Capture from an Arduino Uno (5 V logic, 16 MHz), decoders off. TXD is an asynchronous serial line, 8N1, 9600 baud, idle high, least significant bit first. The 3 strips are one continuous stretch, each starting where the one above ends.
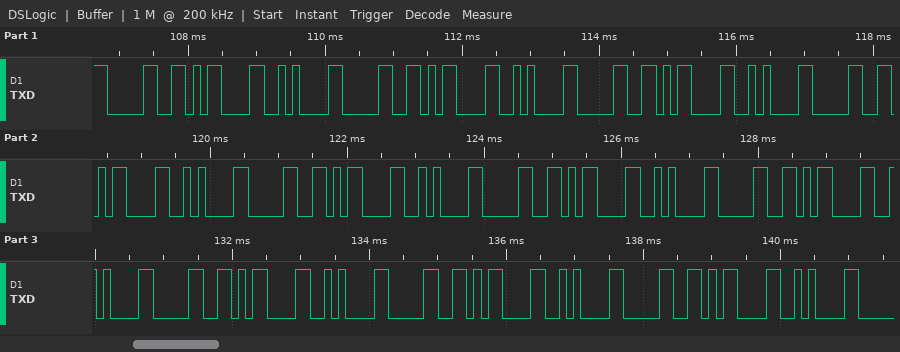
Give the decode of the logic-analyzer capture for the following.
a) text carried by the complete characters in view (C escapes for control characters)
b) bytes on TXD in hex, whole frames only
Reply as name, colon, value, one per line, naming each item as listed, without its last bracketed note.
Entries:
text carried by the complete characters in view: "0\r\n0\r\n0\r\n0\r\n0\r\n0\r\n0\r\n0\r\n0\r\n0\r\n"
bytes on TXD in hex, whole frames only: 30 0D 0A 30 0D 0A 30 0D 0A 30 0D 0A 30 0D 0A 30 0D 0A 30 0D 0A 30 0D 0A 30 0D 0A 30 0D 0A
